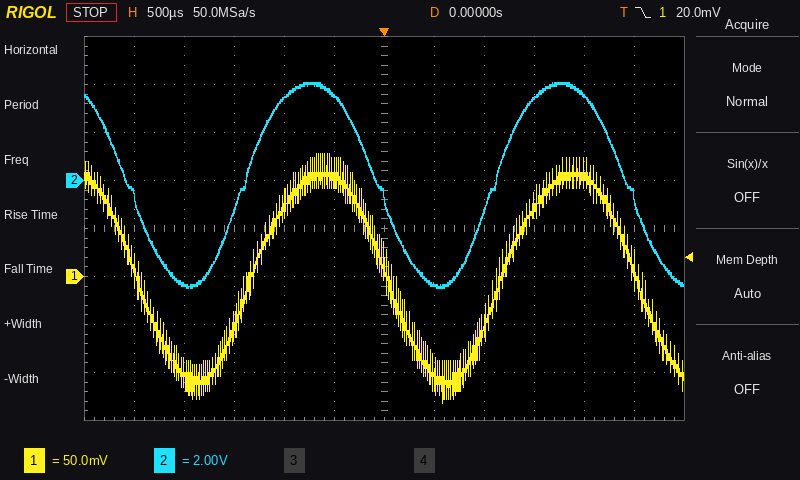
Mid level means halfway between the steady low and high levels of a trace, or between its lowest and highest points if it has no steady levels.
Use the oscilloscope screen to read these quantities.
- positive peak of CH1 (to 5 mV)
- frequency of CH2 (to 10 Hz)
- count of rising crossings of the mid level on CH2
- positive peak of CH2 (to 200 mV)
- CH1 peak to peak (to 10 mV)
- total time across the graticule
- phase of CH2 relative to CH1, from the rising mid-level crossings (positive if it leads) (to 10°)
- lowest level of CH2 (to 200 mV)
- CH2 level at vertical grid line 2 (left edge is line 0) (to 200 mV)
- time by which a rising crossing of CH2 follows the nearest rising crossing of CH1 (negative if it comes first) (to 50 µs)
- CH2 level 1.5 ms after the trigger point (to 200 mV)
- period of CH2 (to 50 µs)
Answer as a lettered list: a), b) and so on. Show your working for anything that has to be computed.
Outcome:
a) 130 mV
b) 1 / 2.50 ms ≈ 400 Hz
c) 2
d) 4.0 V
e) 260 mV
f) 6 ms
g) −360° × (-50 µs) / 2.50 ms ≈ +7.20°, so +10° to the nearest 10°
h) -4.4 V
i) -4.4 V
j) -50 µs
k) 3.4 V
l) 2.50 ms
